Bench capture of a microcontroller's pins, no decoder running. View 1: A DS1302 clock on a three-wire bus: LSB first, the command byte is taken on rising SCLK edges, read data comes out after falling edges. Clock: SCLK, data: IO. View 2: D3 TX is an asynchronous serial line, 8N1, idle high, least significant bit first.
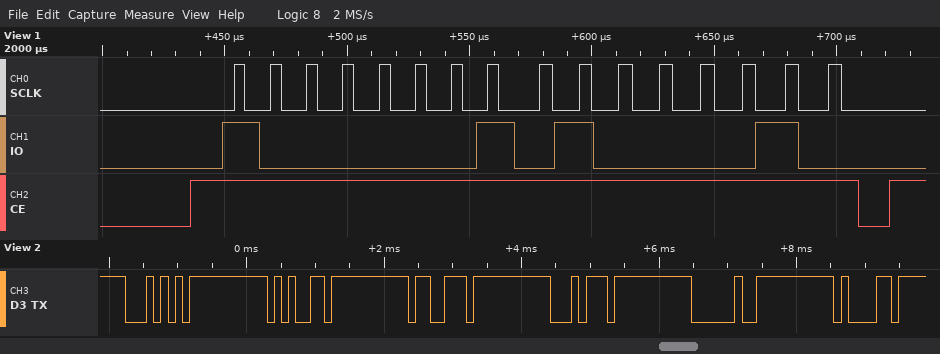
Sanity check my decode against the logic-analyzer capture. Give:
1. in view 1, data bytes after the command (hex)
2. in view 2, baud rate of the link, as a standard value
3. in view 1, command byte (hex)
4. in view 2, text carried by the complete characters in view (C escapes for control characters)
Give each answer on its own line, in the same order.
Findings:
42
9600 baud
0x81
"Test a"
